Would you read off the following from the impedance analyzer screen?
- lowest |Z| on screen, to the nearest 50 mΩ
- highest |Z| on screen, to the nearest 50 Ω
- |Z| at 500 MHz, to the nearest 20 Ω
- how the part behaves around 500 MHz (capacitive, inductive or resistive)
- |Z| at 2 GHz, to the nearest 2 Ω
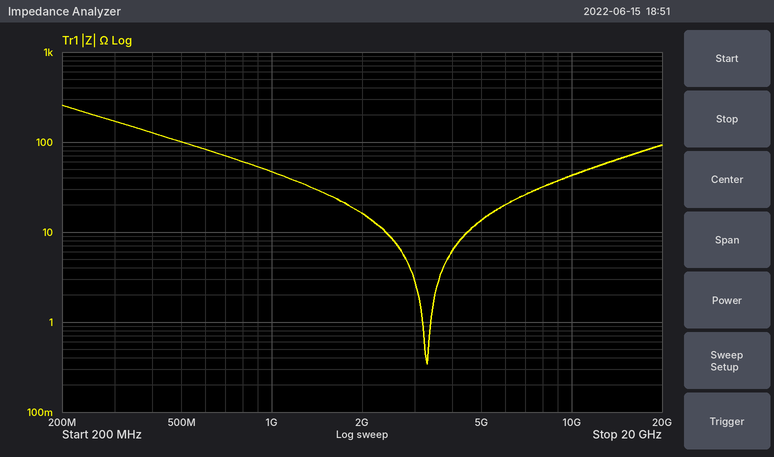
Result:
350 mΩ
250 Ω
100 Ω
capacitive
16 Ω
